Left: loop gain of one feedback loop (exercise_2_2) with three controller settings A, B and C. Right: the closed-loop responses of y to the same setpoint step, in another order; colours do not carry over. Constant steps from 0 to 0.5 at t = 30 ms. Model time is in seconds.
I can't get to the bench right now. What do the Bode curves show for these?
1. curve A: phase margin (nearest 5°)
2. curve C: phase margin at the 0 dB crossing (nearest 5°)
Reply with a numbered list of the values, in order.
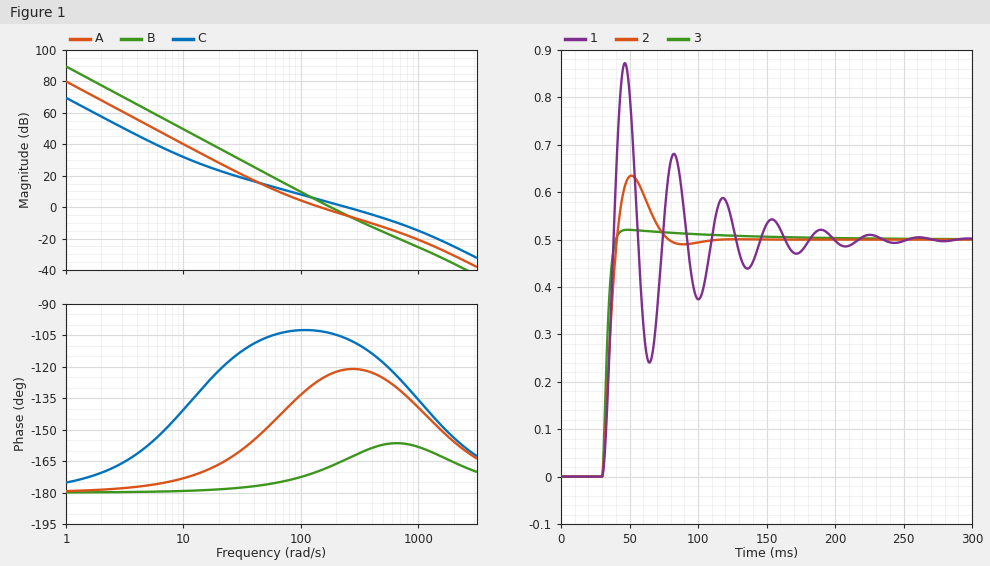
1. 55°
2. 75°
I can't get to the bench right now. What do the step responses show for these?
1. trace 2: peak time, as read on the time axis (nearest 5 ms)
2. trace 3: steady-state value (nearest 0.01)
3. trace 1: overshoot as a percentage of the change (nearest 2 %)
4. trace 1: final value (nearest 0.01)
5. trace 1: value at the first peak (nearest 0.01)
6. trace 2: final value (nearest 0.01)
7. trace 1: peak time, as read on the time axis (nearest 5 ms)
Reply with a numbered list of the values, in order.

1. 50 ms
2. 0.50
3. 74 %
4. 0.50
5. 0.87
6. 0.50
7. 45 ms
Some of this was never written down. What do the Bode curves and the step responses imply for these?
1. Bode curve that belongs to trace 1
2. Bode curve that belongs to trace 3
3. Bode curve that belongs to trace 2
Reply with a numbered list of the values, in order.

1. B
2. C
3. A
